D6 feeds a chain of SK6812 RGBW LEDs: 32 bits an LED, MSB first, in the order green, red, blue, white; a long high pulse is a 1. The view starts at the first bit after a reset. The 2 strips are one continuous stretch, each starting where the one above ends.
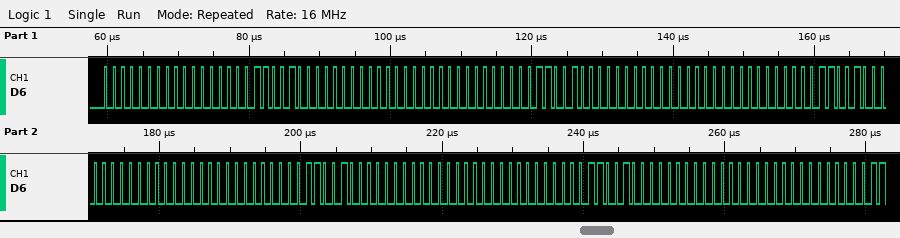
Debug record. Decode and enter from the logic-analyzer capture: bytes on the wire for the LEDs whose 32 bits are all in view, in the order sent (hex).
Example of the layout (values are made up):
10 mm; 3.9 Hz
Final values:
00 00 64 00 00 00 64 00 00 00 64 00 00 00 64 00 00 00 64 00
